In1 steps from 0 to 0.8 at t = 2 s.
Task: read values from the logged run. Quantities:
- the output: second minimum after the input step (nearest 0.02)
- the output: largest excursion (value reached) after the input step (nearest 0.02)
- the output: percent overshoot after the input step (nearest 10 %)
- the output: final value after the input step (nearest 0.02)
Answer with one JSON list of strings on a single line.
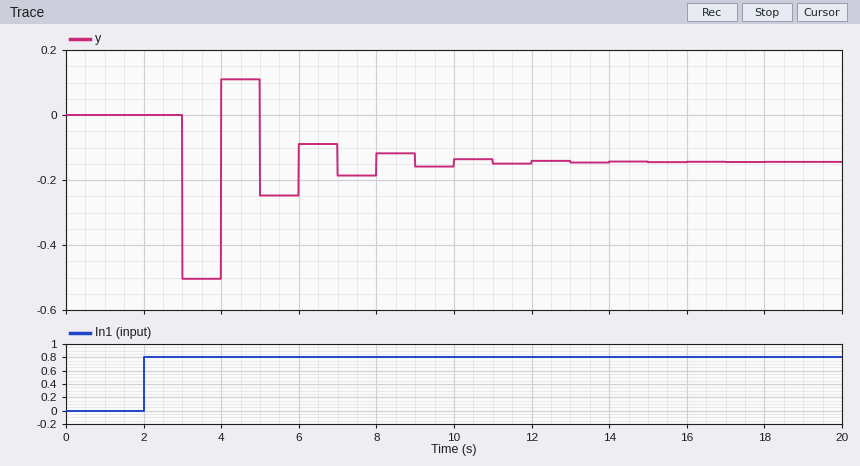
["-0.24", "-0.50", "250 %", "-0.14"]
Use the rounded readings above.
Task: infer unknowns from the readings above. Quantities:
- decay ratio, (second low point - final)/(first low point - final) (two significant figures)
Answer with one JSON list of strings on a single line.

["0.28"]
